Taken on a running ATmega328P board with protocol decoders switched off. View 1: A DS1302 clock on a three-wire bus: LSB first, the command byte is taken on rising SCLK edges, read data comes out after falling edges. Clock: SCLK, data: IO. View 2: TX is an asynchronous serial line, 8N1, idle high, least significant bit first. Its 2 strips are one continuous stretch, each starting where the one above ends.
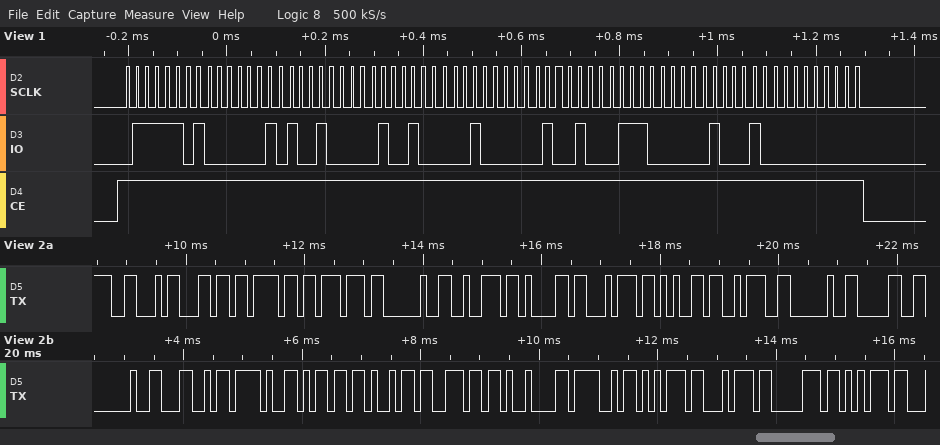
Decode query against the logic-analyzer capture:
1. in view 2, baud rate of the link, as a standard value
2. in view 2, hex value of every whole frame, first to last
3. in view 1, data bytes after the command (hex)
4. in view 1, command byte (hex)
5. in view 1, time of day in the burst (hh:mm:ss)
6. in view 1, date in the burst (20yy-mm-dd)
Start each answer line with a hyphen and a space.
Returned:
- 9600 baud
- 46 6C 6F 77 20 72 61 74 65 3A 20 30 20 4C 2F 6D 69 6E 09 4F 75 74 70 75
- 40 09 12 04 12 07 22 00
- 0xBE
- 12:09:40
- 2022-12-04
